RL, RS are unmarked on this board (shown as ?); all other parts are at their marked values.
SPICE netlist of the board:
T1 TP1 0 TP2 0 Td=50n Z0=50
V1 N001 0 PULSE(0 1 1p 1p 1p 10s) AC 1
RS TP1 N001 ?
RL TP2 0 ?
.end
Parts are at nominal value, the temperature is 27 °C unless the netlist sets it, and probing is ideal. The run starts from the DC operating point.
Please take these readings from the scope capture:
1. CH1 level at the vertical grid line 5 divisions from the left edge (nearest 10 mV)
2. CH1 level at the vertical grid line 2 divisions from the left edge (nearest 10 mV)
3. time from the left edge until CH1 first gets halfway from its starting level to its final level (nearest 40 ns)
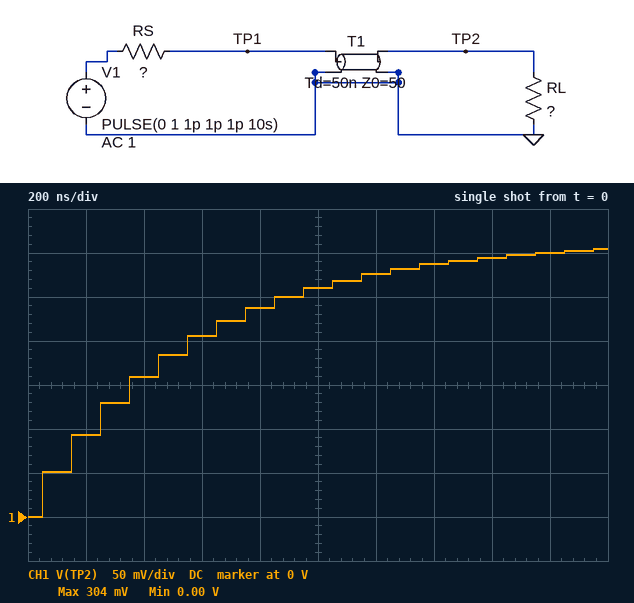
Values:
260 mV
160 mV
360 ns
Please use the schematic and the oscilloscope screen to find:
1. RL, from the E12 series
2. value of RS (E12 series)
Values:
820 Ω
1.8 kΩ
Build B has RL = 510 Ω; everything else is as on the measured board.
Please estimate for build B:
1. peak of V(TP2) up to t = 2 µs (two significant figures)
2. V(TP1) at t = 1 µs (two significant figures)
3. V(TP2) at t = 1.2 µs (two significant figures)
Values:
220 mV
200 mV
210 mV
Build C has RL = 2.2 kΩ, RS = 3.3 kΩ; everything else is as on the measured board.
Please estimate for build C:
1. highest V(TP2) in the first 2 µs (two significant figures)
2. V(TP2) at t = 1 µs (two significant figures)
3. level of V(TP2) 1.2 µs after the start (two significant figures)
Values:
310 mV
210 mV
240 mV
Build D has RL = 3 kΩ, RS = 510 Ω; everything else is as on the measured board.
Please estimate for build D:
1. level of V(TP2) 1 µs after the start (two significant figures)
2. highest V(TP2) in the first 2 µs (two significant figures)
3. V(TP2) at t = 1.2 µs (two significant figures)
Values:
770 mV
850 mV
800 mV
